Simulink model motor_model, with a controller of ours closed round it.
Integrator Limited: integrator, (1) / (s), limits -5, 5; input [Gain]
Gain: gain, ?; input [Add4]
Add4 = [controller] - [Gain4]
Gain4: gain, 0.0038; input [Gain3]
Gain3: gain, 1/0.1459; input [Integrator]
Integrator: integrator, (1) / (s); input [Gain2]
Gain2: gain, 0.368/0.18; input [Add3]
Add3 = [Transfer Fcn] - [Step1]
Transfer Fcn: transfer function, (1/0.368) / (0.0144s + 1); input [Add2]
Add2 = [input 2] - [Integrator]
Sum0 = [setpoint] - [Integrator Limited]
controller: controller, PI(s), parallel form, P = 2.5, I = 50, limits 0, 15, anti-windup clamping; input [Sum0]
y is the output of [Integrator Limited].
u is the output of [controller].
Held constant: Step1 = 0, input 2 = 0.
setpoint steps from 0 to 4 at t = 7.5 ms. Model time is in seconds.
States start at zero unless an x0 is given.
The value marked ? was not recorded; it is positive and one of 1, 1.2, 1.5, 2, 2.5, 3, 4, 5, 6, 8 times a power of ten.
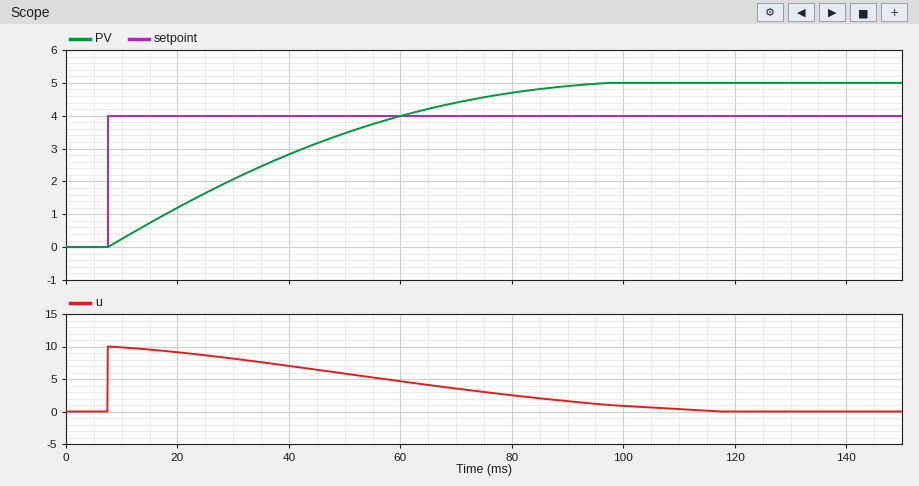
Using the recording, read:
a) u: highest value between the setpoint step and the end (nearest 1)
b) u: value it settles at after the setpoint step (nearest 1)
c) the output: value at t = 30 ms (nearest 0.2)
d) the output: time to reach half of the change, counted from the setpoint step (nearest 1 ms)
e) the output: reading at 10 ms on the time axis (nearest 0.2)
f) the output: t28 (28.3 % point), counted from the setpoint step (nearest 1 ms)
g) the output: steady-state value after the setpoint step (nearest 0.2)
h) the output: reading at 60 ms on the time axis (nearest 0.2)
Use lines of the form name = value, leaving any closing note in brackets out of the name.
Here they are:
u: highest value between the setpoint step and the end = 10
u: value it settles at after the setpoint step = 0
the output: value at t = 30 ms = 2.0
the output: time to reach half of the change, counted from the setpoint step = 28 ms
the output: reading at 10 ms on the time axis = 0.2
the output: t28 (28.3 % point), counted from the setpoint step = 15 ms
the output: steady-state value after the setpoint step = 5.0
the output: reading at 60 ms on the time axis = 4.0
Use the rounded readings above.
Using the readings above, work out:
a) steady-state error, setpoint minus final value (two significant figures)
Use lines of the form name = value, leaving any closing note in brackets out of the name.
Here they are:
steady-state error, setpoint minus final value = -1.0
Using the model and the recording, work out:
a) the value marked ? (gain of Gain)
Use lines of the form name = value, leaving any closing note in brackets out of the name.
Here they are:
the value marked ? = 10
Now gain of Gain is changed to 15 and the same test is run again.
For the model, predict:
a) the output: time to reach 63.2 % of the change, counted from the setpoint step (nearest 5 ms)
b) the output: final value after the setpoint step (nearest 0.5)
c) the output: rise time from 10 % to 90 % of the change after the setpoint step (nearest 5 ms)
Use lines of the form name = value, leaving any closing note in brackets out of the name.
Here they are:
the output: time to reach 63.2 % of the change, counted from the setpoint step = 25 ms
the output: final value after the setpoint step = 5.0
the output: rise time from 10 % to 90 % of the change after the setpoint step = 45 ms
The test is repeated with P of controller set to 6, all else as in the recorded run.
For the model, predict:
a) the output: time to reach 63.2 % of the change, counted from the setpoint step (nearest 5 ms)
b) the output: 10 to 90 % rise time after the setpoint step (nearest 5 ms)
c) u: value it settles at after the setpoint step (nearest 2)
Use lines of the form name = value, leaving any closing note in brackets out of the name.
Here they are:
the output: time to reach 63.2 % of the change, counted from the setpoint step = 20 ms
the output: 10 to 90 % rise time after the setpoint step = 40 ms
u: value it settles at after the setpoint step = 0
